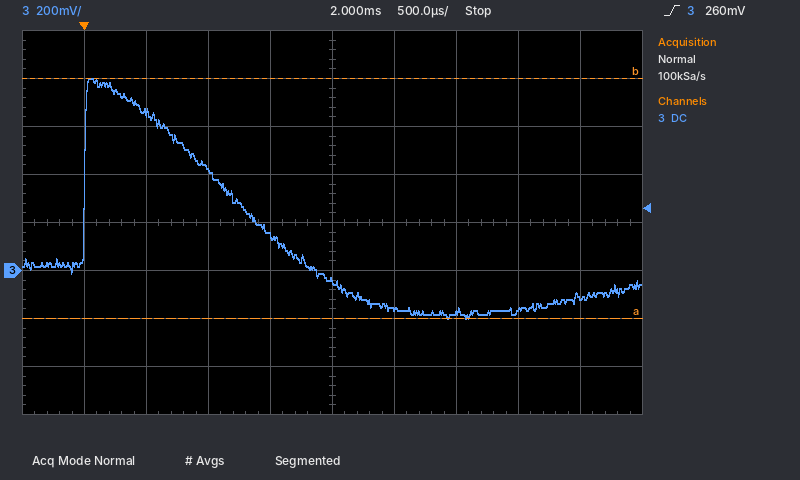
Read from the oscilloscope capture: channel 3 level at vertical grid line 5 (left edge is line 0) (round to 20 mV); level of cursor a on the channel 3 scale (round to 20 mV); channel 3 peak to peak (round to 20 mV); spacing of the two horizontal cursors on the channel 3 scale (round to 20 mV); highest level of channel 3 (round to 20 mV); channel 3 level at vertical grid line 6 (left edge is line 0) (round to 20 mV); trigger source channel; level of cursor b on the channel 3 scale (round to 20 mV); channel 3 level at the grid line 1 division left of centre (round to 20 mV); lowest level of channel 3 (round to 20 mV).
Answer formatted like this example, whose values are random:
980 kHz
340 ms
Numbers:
-40 mV
-200 mV
1.00 V
1.00 V
800 mV
-160 mV
channel 3
800 mV
140 mV
-200 mV
